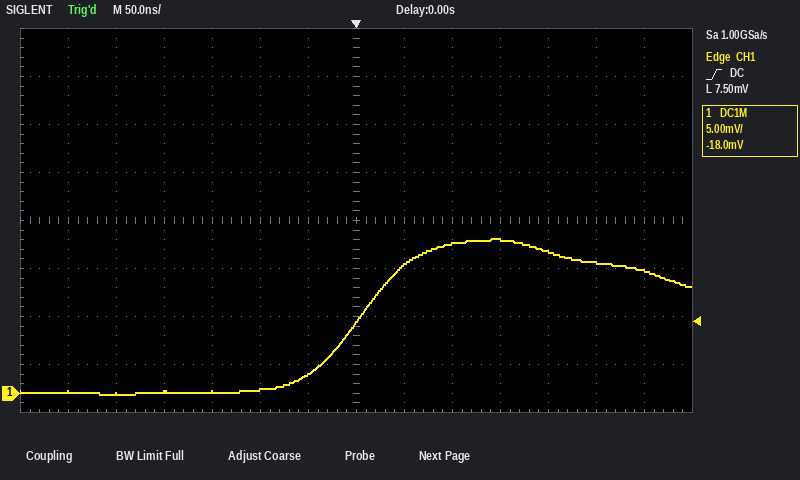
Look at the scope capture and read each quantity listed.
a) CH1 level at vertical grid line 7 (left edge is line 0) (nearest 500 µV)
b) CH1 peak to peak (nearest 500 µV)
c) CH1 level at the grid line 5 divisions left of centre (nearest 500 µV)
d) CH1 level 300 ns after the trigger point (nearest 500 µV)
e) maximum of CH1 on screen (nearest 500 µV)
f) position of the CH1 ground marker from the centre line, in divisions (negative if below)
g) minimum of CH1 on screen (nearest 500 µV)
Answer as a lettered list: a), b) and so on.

a) 7.5 mV
b) 16.0 mV
c) 0.0 mV
d) 13.0 mV
e) 16.0 mV
f) -3.6 div
g) 0.0 mV
